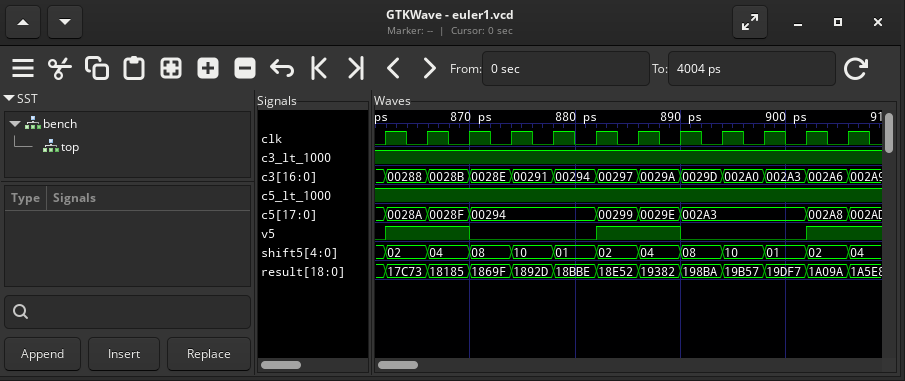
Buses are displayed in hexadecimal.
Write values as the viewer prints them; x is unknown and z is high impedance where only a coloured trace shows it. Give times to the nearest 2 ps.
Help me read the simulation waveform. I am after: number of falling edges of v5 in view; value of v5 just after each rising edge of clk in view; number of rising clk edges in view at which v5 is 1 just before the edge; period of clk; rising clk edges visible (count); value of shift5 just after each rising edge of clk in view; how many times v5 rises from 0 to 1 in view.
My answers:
2
1 1 0 0 0 1 1 0 0 0 1 1
5
4 ps
12
02, 04, 08, 10, 01, 02, 04, 08, 10, 01, 02, 04
3
